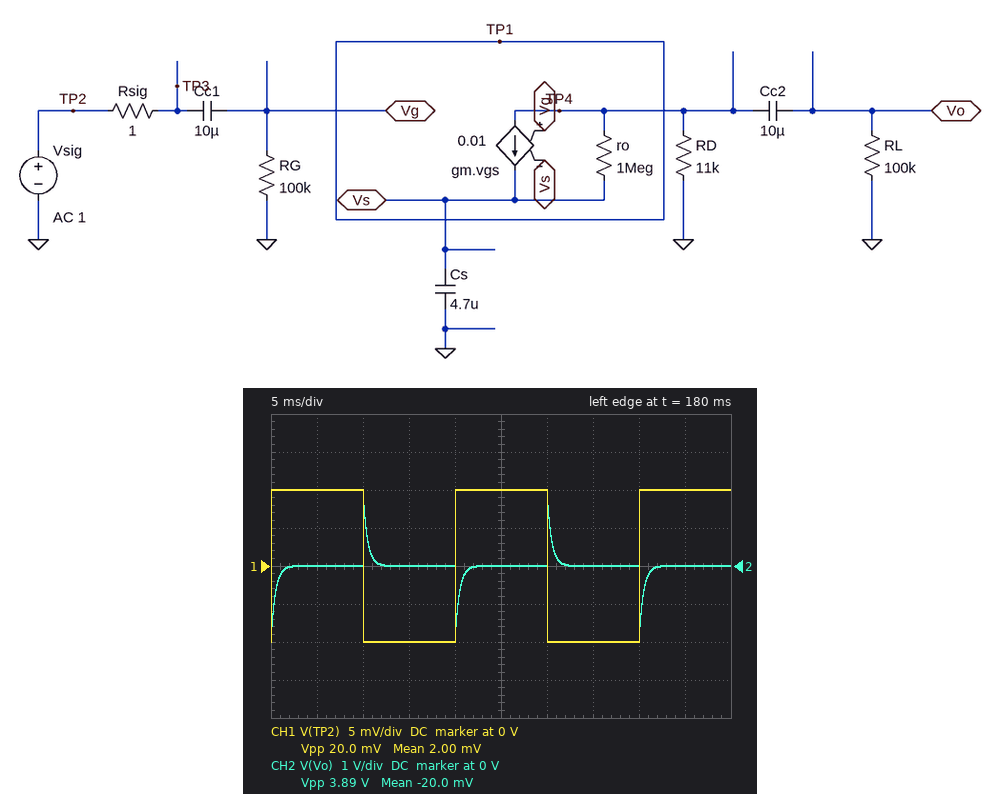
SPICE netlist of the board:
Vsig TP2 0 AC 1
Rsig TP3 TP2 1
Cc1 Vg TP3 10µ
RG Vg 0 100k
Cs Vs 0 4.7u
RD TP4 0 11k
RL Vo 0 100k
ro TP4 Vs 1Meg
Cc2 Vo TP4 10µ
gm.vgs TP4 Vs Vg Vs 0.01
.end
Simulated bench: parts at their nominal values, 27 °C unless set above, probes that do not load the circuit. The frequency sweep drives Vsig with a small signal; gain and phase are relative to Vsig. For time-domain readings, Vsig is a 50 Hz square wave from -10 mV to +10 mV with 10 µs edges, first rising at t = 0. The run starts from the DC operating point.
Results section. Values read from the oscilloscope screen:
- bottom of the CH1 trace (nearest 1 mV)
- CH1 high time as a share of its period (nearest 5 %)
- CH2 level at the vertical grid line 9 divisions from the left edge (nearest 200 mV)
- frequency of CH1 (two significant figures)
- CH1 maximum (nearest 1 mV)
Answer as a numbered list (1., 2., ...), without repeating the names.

1. -10 mV
2. 50 %
3. 0 V
4. 50 Hz
5. 10 mV
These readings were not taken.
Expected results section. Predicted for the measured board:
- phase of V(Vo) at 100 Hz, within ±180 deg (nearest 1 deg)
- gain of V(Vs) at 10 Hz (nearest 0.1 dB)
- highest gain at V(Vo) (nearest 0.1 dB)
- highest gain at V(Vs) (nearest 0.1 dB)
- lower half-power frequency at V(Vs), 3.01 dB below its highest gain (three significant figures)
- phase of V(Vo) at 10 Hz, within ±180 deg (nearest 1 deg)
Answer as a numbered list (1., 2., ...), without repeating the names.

1. -106 deg
2. 0 dB
3. 39.8 dB
4. 0 dB
5. 159 mHz
6. -90 deg
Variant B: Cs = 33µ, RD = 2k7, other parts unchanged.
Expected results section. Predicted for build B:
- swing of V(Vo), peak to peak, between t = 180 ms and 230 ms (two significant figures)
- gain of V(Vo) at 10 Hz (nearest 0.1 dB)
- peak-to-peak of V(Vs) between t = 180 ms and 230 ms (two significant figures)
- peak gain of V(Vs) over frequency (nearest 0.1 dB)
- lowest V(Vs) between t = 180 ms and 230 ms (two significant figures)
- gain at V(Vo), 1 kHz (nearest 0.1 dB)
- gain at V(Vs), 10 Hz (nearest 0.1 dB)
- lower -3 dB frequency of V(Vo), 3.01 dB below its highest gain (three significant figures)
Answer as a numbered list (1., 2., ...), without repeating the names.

1. 1.0 V
2. 14.5 dB
3. 18 mV
4. 0 dB
5. -1.0 mV
6. 28.4 dB
7. -0.2 dB
8. 48.1 Hz
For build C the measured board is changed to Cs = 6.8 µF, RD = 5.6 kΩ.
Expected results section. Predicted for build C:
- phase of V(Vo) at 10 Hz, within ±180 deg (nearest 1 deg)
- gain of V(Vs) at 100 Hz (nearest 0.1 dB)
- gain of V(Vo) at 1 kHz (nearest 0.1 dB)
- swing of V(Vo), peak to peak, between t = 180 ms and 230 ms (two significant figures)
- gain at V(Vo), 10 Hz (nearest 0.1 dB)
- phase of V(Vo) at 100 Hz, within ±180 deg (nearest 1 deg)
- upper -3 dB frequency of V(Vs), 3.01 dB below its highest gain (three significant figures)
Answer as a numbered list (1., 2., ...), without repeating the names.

1. -91 deg
2. -0.7 dB
3. 34.2 dB
4. 2.1 V
5. 7.1 dB
6. -113 deg
7. 233 Hz
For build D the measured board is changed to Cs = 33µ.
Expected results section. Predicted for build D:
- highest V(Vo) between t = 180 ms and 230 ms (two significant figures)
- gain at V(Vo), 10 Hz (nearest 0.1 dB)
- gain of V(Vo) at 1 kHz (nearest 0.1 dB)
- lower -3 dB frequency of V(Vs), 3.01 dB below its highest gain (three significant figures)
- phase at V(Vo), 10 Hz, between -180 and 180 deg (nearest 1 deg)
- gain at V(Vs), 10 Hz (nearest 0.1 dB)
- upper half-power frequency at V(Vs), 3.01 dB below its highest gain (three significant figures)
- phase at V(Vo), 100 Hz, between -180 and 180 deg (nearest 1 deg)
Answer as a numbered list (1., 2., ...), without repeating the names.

1. 1.9 V
2. 26.1 dB
3. 39.8 dB
4. 158 mHz
5. -100 deg
6. -0.2 dB
7. 48.1 Hz
8. -154 deg
